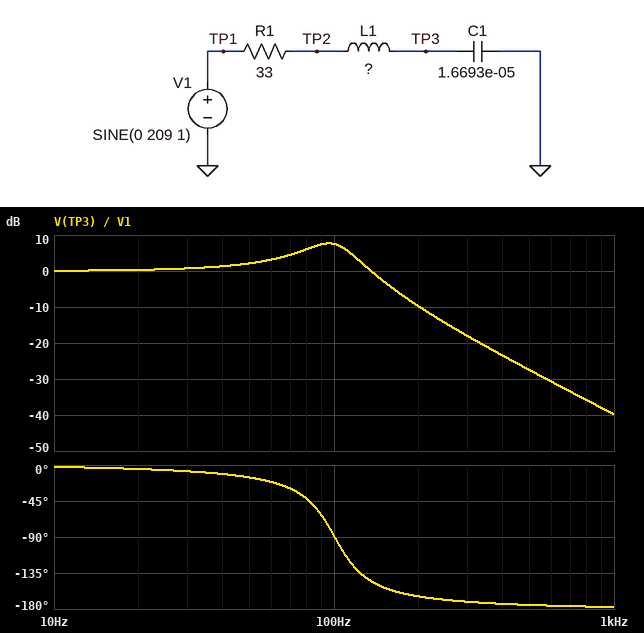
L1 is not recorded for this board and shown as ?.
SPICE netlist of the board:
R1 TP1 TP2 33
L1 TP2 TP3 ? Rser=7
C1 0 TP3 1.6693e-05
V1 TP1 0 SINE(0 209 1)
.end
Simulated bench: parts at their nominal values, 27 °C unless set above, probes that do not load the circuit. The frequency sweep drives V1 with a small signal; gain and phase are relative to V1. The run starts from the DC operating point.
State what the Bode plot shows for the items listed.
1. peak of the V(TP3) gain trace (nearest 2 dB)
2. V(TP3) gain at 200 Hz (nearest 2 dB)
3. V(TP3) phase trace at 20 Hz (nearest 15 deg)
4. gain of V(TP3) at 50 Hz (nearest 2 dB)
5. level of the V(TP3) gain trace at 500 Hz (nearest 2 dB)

8 dB
-10 dB
0 deg
2 dB
-28 dB
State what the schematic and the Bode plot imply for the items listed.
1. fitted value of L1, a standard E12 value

150 mH
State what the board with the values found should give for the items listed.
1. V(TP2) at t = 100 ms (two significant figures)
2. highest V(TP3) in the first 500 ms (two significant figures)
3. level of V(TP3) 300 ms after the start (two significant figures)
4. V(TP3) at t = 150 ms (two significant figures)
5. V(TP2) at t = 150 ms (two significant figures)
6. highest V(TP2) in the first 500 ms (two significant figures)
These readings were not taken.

120 V
210 V
200 V
170 V
170 V
210 V
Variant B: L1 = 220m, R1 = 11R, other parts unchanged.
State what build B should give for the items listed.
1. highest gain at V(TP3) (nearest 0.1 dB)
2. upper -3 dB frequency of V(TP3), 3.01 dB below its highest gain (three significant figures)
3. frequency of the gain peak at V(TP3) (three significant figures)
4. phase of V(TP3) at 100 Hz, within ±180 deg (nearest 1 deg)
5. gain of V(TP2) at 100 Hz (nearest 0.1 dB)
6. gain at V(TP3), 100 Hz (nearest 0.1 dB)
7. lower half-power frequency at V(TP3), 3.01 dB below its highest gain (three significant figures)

16.1 dB
88.8 Hz
82.5 Hz
-157 deg
-0.6 dB
6.2 dB
75.7 Hz
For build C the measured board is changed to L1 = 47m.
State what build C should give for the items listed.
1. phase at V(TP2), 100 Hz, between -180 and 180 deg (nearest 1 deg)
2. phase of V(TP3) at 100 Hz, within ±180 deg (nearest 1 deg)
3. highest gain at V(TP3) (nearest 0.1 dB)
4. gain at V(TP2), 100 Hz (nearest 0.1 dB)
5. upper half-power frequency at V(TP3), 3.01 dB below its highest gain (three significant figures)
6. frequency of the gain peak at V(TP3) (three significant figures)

-25 deg
-31 deg
3.1 dB
-1.3 dB
214 Hz
152 Hz
